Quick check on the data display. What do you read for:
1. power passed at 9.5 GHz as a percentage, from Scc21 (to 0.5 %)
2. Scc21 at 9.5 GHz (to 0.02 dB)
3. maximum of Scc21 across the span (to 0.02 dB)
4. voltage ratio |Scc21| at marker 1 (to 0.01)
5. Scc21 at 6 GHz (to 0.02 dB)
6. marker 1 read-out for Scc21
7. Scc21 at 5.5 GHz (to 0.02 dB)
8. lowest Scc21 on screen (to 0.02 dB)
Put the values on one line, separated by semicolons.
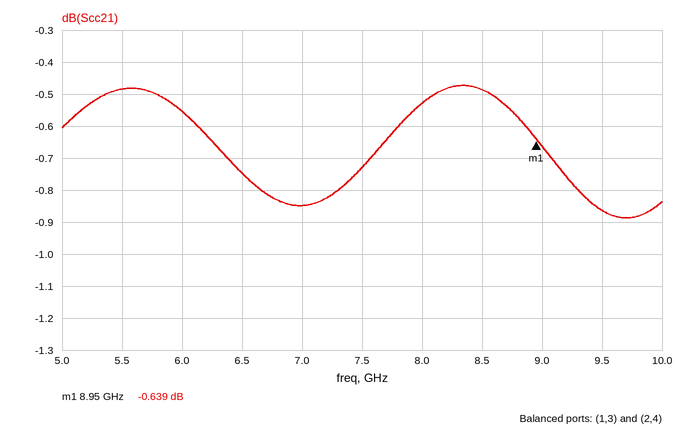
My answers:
82.0 %; -0.86 dB; -0.48 dB; 0.93; -0.56 dB; -0.639 dB; -0.48 dB; -0.88 dB
